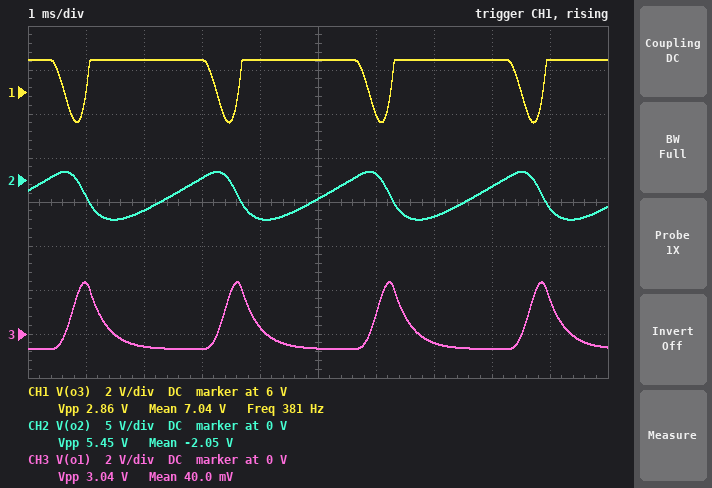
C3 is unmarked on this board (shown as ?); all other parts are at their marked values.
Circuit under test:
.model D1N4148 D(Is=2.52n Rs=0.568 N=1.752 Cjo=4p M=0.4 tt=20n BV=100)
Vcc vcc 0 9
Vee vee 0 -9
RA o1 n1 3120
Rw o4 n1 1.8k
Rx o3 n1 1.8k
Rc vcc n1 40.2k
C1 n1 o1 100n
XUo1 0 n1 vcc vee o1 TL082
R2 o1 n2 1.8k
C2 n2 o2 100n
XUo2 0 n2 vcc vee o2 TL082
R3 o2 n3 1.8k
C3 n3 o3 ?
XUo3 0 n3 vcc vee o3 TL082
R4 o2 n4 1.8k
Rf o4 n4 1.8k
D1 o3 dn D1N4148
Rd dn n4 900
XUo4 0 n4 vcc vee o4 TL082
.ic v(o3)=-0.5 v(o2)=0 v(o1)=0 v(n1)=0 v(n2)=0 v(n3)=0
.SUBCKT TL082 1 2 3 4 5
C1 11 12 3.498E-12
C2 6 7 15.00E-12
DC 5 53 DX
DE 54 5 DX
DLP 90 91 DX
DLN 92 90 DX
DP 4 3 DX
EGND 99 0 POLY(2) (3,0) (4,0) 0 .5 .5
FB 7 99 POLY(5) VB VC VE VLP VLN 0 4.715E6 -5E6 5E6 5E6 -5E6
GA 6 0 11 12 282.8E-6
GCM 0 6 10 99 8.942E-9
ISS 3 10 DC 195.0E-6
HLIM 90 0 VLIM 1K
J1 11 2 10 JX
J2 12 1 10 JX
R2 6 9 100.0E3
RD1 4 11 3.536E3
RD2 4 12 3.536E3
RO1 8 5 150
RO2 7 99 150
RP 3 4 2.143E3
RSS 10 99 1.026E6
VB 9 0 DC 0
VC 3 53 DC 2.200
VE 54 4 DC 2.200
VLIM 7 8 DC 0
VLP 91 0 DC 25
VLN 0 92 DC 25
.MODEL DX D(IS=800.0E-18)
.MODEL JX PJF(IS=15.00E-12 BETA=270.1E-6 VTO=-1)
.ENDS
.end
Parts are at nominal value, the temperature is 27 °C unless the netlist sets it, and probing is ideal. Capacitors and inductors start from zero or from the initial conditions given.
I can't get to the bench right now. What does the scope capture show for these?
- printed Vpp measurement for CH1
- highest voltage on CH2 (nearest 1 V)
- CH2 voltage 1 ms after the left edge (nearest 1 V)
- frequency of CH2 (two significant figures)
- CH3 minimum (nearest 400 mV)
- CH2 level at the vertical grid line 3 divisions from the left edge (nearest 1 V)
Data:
2.86 V
1 V
-2 V
380 Hz
-800 mV
0 V
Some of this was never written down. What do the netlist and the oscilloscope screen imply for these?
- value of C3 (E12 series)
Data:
56 nF
